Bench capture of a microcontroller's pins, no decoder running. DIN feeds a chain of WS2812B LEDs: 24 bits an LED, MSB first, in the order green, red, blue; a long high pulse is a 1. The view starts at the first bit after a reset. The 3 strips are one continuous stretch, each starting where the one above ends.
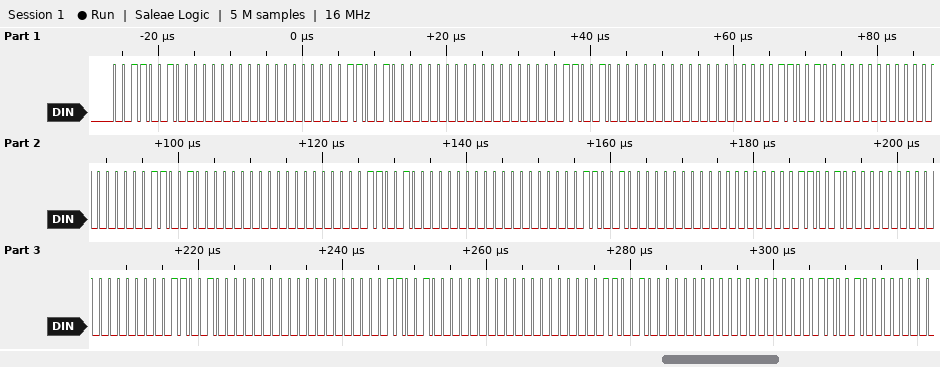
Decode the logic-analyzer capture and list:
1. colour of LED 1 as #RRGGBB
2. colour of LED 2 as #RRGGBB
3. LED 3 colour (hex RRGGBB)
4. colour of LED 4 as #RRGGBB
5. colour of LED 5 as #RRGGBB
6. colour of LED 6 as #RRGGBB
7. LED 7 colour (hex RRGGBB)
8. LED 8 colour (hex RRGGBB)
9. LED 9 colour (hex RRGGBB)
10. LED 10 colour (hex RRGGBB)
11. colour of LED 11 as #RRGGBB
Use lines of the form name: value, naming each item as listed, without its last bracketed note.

colour of LED 1 as #RRGGBB: #003200
colour of LED 2 as #RRGGBB: #003200
LED 3 colour: #003200
colour of LED 4 as #RRGGBB: #003200
colour of LED 5 as #RRGGBB: #003200
colour of LED 6 as #RRGGBB: #003200
LED 7 colour: #003200
LED 8 colour: #003200
LED 9 colour: #003200
LED 10 colour: #003200
colour of LED 11 as #RRGGBB: #003200
